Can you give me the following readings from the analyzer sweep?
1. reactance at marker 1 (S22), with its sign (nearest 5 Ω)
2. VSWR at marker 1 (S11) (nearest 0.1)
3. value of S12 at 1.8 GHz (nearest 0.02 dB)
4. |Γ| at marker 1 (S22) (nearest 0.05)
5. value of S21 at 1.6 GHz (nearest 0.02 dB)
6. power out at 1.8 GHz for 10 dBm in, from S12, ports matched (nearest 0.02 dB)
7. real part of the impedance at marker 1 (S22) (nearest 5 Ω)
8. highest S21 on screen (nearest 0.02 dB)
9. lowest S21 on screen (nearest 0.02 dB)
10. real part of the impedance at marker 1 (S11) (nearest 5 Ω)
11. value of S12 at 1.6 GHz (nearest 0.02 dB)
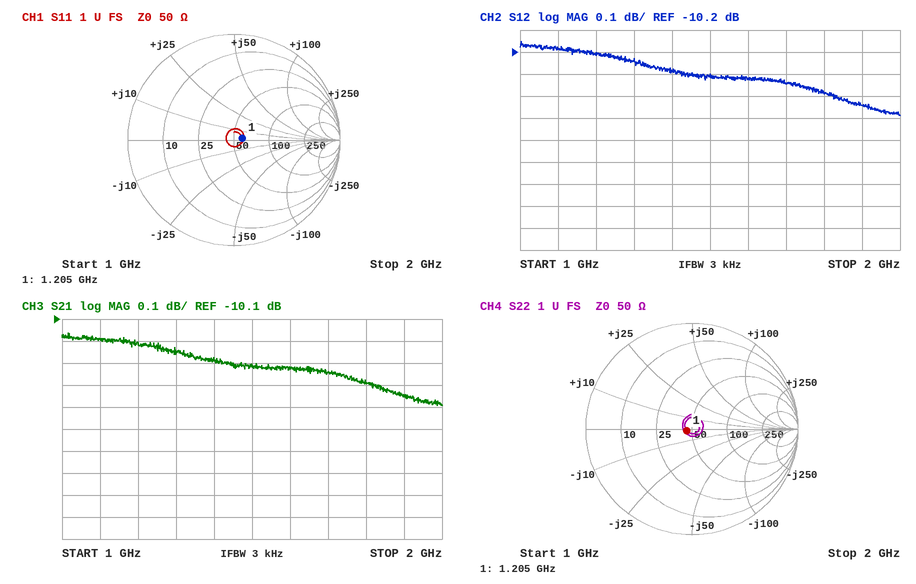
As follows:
0 Ω
1.2
-10.38 dB
0.05
-10.32 dB
-0.38 dBm
45 Ω
-10.16 dB
-10.50 dB
60 Ω
-10.32 dB
